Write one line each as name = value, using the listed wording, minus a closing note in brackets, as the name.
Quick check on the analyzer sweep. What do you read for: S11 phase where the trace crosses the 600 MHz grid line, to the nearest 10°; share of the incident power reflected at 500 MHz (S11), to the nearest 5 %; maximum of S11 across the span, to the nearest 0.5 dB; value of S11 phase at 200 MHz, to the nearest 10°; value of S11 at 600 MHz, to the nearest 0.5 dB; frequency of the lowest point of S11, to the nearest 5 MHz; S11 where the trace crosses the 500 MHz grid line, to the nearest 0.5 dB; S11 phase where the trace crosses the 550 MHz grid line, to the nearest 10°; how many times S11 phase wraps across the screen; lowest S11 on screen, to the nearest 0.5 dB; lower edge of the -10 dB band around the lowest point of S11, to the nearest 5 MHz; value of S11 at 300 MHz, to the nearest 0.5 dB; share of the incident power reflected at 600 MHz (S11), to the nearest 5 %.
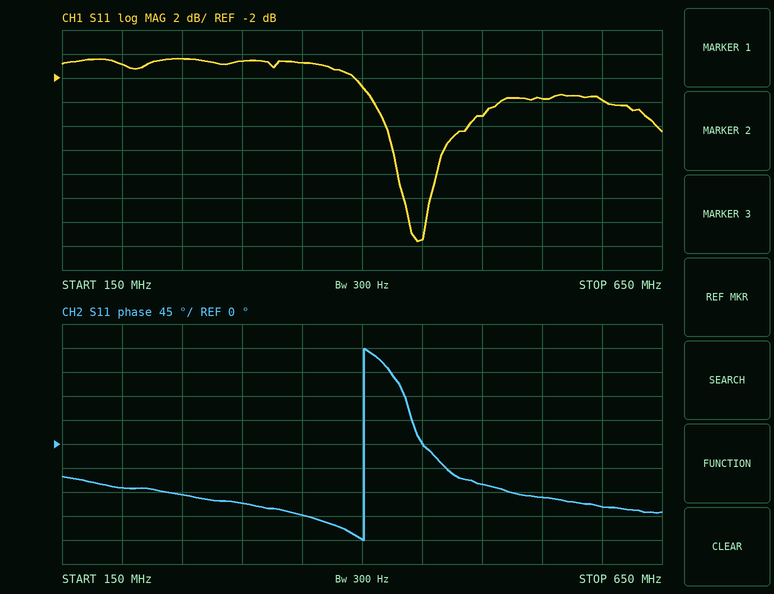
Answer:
S11 phase where the trace crosses the 600 MHz grid line, to the nearest 10° = -120°
share of the incident power reflected at 500 MHz (S11), to the nearest 5 % = 30 %
maximum of S11 across the span, to the nearest 0.5 dB = -0.5 dB
value of S11 phase at 200 MHz, to the nearest 10° = -80°
value of S11 at 600 MHz, to the nearest 0.5 dB = -4.0 dB
frequency of the lowest point of S11, to the nearest 5 MHz = 445 MHz
S11 where the trace crosses the 500 MHz grid line, to the nearest 0.5 dB = -5.0 dB
S11 phase where the trace crosses the 550 MHz grid line, to the nearest 10° = -100°
how many times S11 phase wraps across the screen = 1
lowest S11 on screen, to the nearest 0.5 dB = -15.5 dB
lower edge of the -10 dB band around the lowest point of S11, to the nearest 5 MHz = 430 MHz
value of S11 at 300 MHz, to the nearest 0.5 dB = -0.5 dB
share of the incident power reflected at 600 MHz (S11), to the nearest 5 % = 40 %
